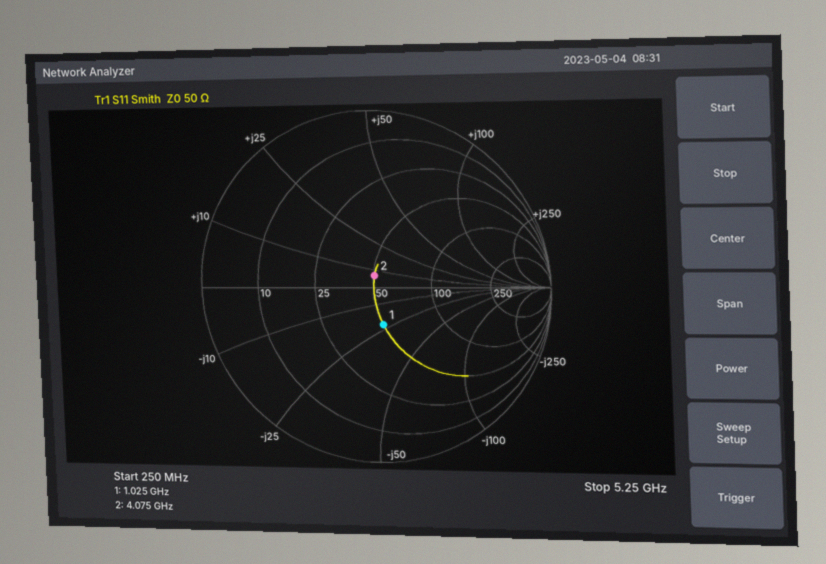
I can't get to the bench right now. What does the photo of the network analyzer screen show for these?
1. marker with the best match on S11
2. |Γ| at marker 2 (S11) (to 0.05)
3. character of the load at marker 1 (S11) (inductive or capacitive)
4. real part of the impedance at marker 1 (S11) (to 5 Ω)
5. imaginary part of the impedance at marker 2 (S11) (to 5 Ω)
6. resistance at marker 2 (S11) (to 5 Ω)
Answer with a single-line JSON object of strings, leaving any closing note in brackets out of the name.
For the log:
{"marker with the best match on S11": "marker 2", "|Γ| at marker 2 (S11)": "0.05", "character of the load at marker 1 (S11)": "capacitive", "real part of the impedance at marker 1 (S11)": "50 Ω", "imaginary part of the impedance at marker 2 (S11)": "+5 Ω", "resistance at marker 2 (S11)": "50 Ω"}
